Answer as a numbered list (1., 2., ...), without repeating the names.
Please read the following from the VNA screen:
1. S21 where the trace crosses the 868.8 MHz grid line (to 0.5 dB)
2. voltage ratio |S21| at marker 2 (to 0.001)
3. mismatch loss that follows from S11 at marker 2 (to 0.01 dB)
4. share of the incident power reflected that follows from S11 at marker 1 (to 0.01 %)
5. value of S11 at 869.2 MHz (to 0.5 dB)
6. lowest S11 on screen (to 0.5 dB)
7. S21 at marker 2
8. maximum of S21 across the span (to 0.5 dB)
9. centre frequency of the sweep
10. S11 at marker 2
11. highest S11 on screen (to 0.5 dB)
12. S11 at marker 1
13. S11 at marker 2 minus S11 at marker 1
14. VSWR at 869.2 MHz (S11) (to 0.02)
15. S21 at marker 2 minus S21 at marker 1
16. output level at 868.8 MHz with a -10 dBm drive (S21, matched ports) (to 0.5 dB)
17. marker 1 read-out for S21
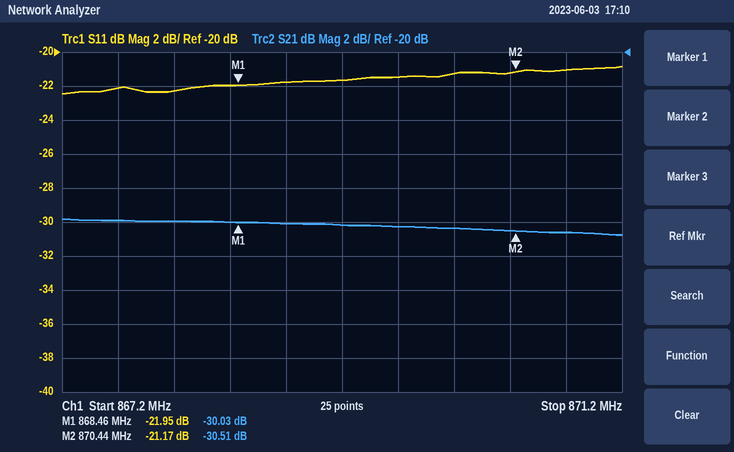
1. -30.0 dB
2. 0.030
3. 0.03 dB
4. 0.64 %
5. -21.5 dB
6. -22.5 dB
7. -30.51 dB
8. -30.0 dB
9. 869.2 MHz
10. -21.17 dB
11. -21.0 dB
12. -21.95 dB
13. 0.78 dB
14. 1.18
15. -0.48 dB
16. -40.0 dBm
17. -30.03 dB
